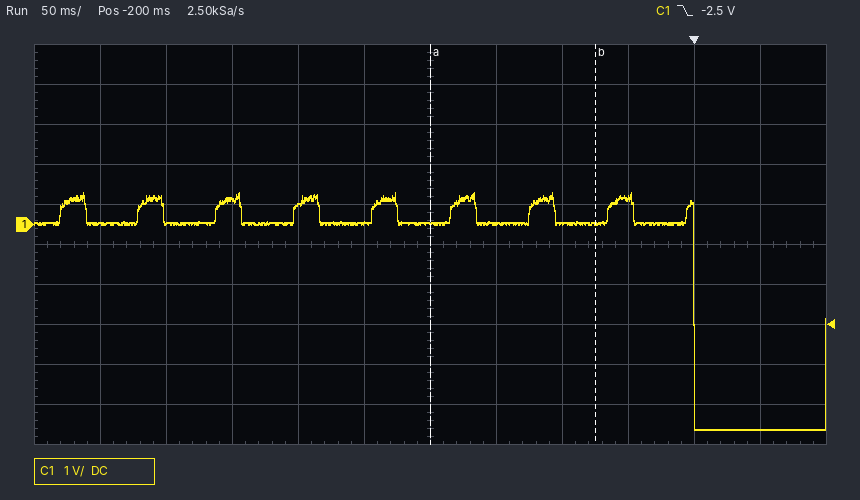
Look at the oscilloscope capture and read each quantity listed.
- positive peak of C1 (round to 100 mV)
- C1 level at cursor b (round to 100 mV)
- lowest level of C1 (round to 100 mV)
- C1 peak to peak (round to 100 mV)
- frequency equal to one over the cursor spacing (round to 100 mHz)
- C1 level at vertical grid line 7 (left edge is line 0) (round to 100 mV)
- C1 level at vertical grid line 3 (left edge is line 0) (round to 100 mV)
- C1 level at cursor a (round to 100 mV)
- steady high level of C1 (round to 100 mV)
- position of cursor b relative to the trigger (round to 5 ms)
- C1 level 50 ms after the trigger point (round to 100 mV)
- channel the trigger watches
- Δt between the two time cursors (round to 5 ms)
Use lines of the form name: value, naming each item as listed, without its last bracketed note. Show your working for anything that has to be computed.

positive peak of C1: 800 mV
C1 level at cursor b: 0.0 V
lowest level of C1: -5.1 V
C1 peak to peak: 800 mV − (-5.1 V) = 5.9 V
frequency equal to one over the cursor spacing: 1 / 125 ms ≈ 8.0 Hz
C1 level at vertical grid line 7 (left edge is line 0): 0.0 V
C1 level at vertical grid line 3 (left edge is line 0): 600 mV
C1 level at cursor a: 0.0 V
steady high level of C1: 0.0 V
position of cursor b relative to the trigger: -75 ms
C1 level 50 ms after the trigger point: -5.1 V
channel the trigger watches: C1
Δt between the two time cursors: 125 ms
